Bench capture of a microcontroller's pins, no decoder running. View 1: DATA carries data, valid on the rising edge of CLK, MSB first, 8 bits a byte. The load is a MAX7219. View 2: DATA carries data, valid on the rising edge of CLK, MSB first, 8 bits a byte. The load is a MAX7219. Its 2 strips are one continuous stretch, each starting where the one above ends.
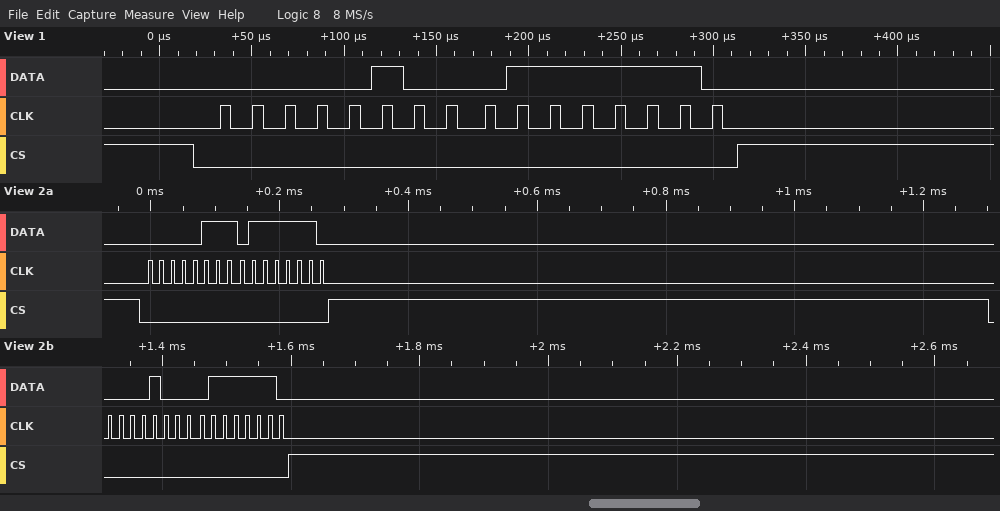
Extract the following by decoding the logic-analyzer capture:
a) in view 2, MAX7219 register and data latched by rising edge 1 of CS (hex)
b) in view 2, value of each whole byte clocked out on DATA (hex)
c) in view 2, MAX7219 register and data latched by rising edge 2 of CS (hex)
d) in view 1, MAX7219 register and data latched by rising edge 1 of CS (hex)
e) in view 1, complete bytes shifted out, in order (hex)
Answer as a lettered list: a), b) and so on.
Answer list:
a) register 0x7, data 0x7E
b) 07 7E 08 7E
c) register 0x8, data 0x7E
d) register 0x4, data 0x7E
e) 04 7E
